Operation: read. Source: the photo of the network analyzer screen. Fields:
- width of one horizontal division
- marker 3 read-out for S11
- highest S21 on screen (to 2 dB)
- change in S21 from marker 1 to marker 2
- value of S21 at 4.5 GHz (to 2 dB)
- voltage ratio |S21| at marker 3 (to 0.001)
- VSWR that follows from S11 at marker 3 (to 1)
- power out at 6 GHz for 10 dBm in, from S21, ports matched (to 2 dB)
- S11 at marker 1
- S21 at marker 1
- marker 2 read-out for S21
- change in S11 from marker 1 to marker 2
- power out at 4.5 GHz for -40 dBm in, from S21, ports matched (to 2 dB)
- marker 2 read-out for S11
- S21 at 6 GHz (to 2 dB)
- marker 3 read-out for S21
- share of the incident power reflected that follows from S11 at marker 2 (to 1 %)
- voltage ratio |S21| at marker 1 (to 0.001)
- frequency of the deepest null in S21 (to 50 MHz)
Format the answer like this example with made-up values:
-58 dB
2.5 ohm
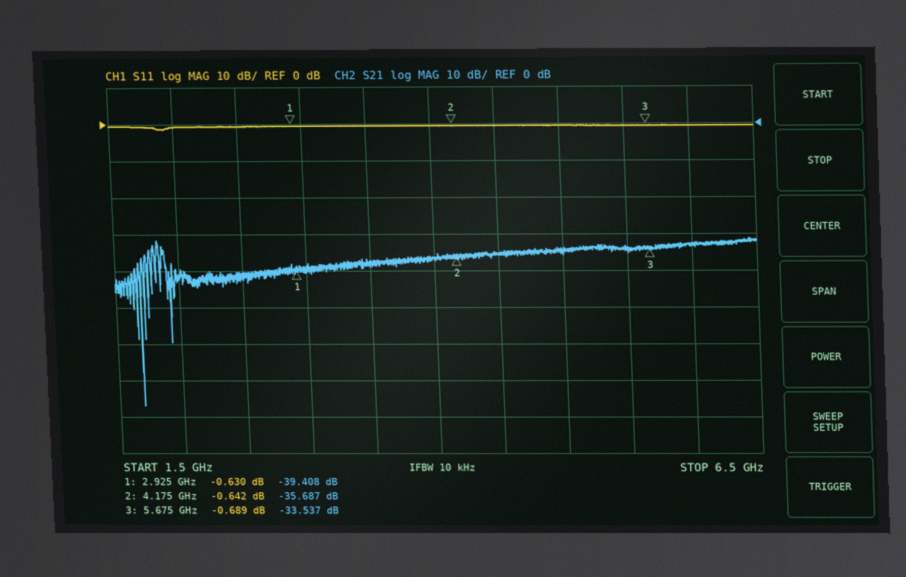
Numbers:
500 MHz
-0.689 dB
-32 dB
3.721 dB
-36 dB
0.021
25
-22 dBm
-0.630 dB
-39.408 dB
-35.687 dB
-0.012 dB
-76 dBm
-0.642 dB
-32 dB
-33.537 dB
86 %
0.011
1.70 GHz
